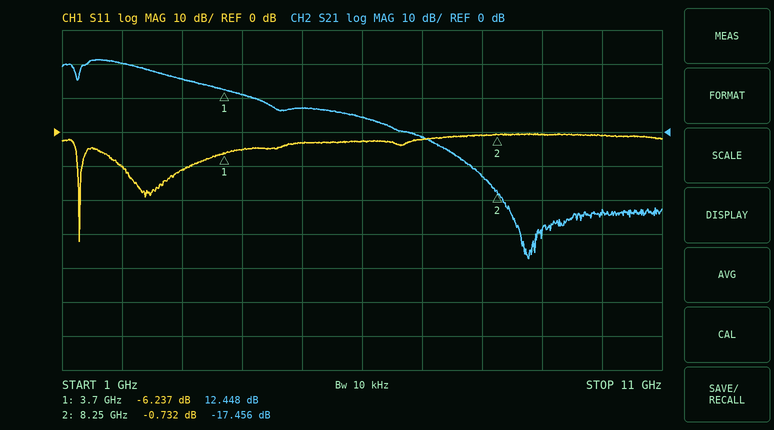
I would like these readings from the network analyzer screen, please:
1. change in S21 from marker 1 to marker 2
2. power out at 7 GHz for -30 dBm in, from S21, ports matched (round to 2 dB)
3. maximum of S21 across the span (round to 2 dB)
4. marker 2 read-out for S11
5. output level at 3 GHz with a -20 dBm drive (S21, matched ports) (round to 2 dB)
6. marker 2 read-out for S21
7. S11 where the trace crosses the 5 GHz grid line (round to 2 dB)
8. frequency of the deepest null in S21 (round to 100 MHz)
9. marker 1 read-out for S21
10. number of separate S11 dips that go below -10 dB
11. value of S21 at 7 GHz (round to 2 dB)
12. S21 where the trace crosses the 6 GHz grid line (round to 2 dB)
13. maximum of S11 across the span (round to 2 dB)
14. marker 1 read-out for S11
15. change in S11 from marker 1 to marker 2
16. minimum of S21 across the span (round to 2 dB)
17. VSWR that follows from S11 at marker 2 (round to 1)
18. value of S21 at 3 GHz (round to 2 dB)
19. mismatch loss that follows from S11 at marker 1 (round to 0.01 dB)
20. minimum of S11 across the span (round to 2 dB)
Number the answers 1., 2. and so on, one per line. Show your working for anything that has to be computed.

1. -17.456 − (12.448) = -29.904 dB
2. -30 dBm + (-2 dB) = -32 dBm
3. 22 dB
4. -0.732 dB
5. -20 dBm + (16 dB) = -4 dBm
6. -17.456 dB
7. -4 dB
8. 8.8 GHz
9. 12.448 dB
10. 2
11. -2 dB
12. 4 dB
13. 0 dB
14. -6.237 dB
15. -0.732 − (-6.237) = 5.505 dB
16. -38 dB
17. (1 + 0.9192)/(1 − 0.9192) ≈ 24
18. 16 dB
19. −10 log10(1 − 10^(-6.237/10)) ≈ 1.18 dB
20. -32 dB
